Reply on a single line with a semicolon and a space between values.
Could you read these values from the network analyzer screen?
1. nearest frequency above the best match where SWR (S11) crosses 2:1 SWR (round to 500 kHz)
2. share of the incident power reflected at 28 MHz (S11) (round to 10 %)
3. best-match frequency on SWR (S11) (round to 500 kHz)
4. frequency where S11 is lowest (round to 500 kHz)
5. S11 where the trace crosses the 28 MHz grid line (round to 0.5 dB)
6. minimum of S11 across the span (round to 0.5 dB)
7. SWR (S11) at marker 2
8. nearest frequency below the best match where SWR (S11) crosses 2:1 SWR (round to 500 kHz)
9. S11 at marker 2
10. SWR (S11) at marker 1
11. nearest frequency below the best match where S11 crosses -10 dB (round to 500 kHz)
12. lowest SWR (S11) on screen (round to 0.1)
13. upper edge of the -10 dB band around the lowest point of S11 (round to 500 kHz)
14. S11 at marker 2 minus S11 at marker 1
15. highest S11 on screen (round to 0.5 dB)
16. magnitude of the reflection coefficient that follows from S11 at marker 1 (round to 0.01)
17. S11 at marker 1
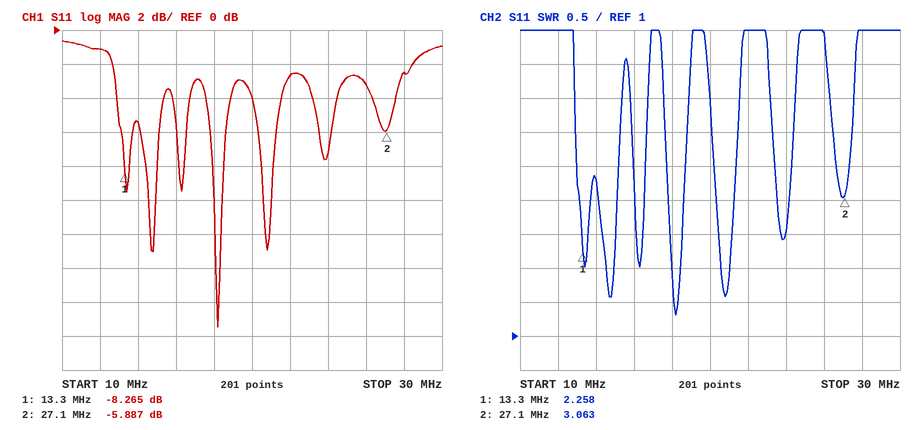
18.5 MHz; 60 %; 18.0 MHz; 18.0 MHz; -2.5 dB; -17.5 dB; 3.063; 18.0 MHz; -5.887 dB; 2.258; 18.0 MHz; 1.3; 18.5 MHz; 2.378 dB; -0.5 dB; 0.39; -8.265 dB
